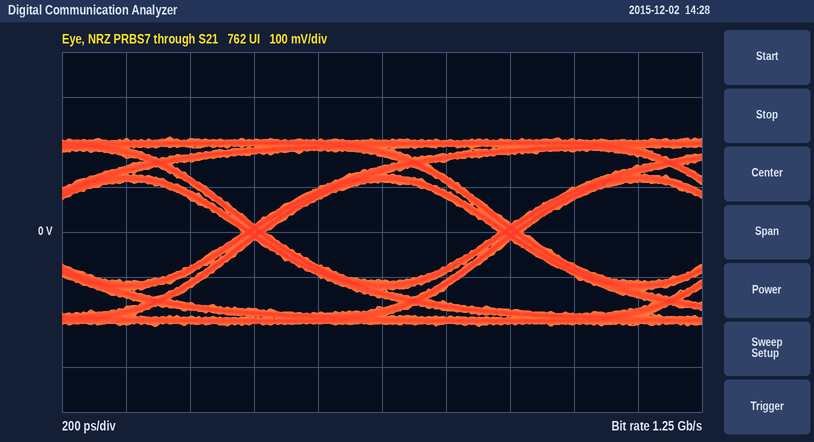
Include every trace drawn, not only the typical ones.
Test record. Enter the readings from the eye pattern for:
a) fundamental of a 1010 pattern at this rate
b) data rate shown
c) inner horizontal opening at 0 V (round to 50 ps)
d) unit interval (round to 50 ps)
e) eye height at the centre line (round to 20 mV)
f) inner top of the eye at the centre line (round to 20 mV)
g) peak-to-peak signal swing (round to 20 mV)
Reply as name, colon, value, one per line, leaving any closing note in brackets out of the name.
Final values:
fundamental of a 1010 pattern at this rate: 625 MHz
data rate shown: 1.25 Gb/s
inner horizontal opening at 0 V: 750 ps
unit interval: 800 ps
eye height at the centre line: 220 mV
inner top of the eye at the centre line: 120 mV
peak-to-peak signal swing: 420 mV
